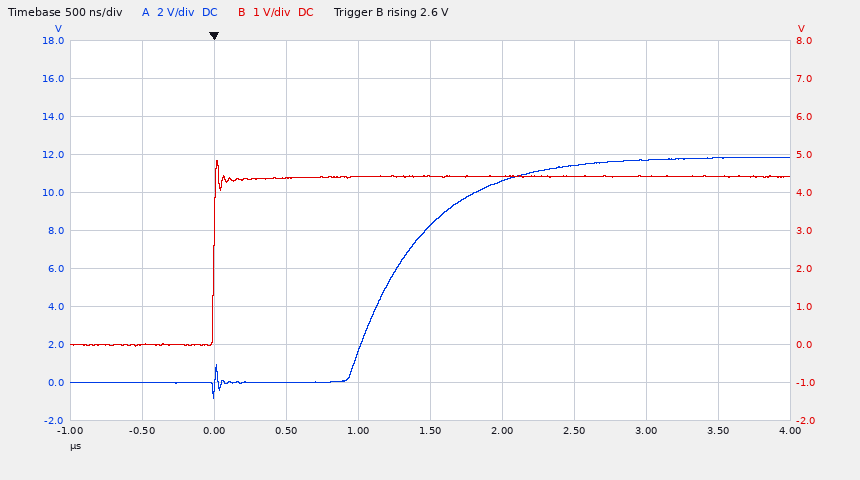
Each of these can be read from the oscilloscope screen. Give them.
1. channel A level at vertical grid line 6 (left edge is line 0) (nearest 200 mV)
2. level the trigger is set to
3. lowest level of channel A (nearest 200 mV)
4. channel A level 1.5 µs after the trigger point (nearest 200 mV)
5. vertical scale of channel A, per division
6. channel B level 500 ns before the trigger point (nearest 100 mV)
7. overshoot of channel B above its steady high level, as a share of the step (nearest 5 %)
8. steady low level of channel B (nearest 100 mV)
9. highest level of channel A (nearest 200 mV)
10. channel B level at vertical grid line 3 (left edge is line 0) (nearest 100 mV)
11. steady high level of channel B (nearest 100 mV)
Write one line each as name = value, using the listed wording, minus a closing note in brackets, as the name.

channel A level at vertical grid line 6 (left edge is line 0) = 10.6 V
level the trigger is set to = 2.6 V
lowest level of channel A = -800 mV
channel A level 1.5 µs after the trigger point = 8.2 V
vertical scale of channel A, per division = 2 V
channel B level 500 ns before the trigger point = 0.0 V
overshoot of channel B above its steady high level, as a share of the step = 10 %
steady low level of channel B = 0.0 V
highest level of channel A = 11.8 V
channel B level at vertical grid line 3 (left edge is line 0) = 4.4 V
steady high level of channel B = 4.4 V
